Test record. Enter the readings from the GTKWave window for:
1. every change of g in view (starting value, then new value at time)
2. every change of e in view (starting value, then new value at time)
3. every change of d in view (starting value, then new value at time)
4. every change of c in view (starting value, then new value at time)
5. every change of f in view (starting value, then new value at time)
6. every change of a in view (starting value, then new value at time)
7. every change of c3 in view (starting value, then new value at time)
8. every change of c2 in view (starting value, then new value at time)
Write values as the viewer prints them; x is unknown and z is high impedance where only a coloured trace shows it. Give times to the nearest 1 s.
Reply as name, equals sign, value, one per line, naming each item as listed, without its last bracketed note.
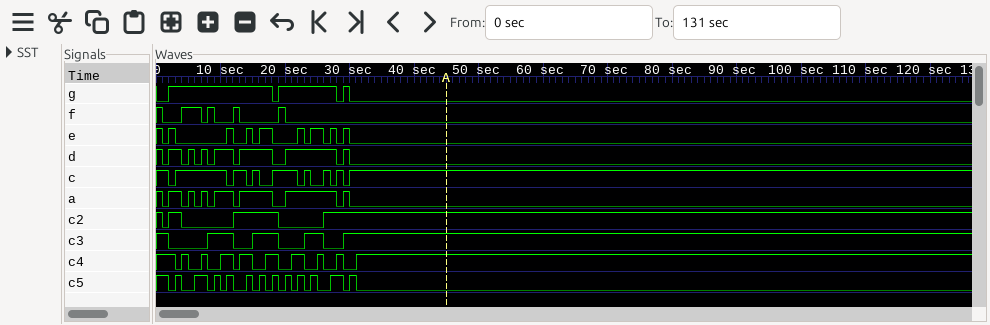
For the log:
every change of g in view = 0, 1 at 2 s, 0 at 18 s, 1 at 19 s, 0 at 28 s, 1 at 29 s, 0 at 30 s
every change of e in view = 1, 0 at 1 s, 1 at 2 s, 0 at 3 s, 1 at 11 s, 0 at 12 s, 1 at 14 s, 0 at 15 s, 1 at 16 s, 0 at 18 s, 1 at 22 s, 0 at 23 s, 1 at 24 s, 0 at 26 s, 1 at 27 s, 0 at 28 s, 1 at 29 s, 0 at 30 s
every change of d in view = 1, 0 at 1 s, 1 at 2 s, 0 at 4 s, 1 at 5 s, 0 at 6 s, 1 at 7 s, 0 at 8 s, 1 at 9 s, 0 at 12 s, 1 at 13 s, 0 at 18 s, 1 at 20 s, 0 at 28 s, 1 at 29 s, 0 at 30 s
every change of c in view = 1, 0 at 2 s, 1 at 3 s, 0 at 11 s, 1 at 12 s, 0 at 14 s, 1 at 15 s, 0 at 16 s, 1 at 18 s, 0 at 22 s, 1 at 23 s, 0 at 24 s, 1 at 26 s, 0 at 27 s, 1 at 28 s, 0 at 29 s, 1 at 30 s
every change of f in view = 1, 0 at 1 s, 1 at 4 s, 0 at 7 s, 1 at 8 s, 0 at 9 s, 1 at 12 s, 0 at 13 s, 1 at 19 s, 0 at 20 s
every change of a in view = 1, 0 at 1 s, 1 at 2 s, 0 at 4 s, 1 at 5 s, 0 at 6 s, 1 at 7 s, 0 at 8 s, 1 at 9 s, 0 at 12 s, 1 at 13 s, 0 at 18 s, 1 at 20 s, 0 at 28 s, 1 at 29 s, 0 at 30 s
every change of c3 in view = 1, 0 at 2 s, 1 at 8 s, 0 at 12 s, 1 at 15 s, 0 at 19 s, 1 at 23 s, 0 at 26 s, 1 at 29 s
every change of c2 in view = 1, 0 at 1 s, 1 at 2 s, 0 at 4 s, 1 at 12 s, 0 at 19 s, 1 at 26 s
